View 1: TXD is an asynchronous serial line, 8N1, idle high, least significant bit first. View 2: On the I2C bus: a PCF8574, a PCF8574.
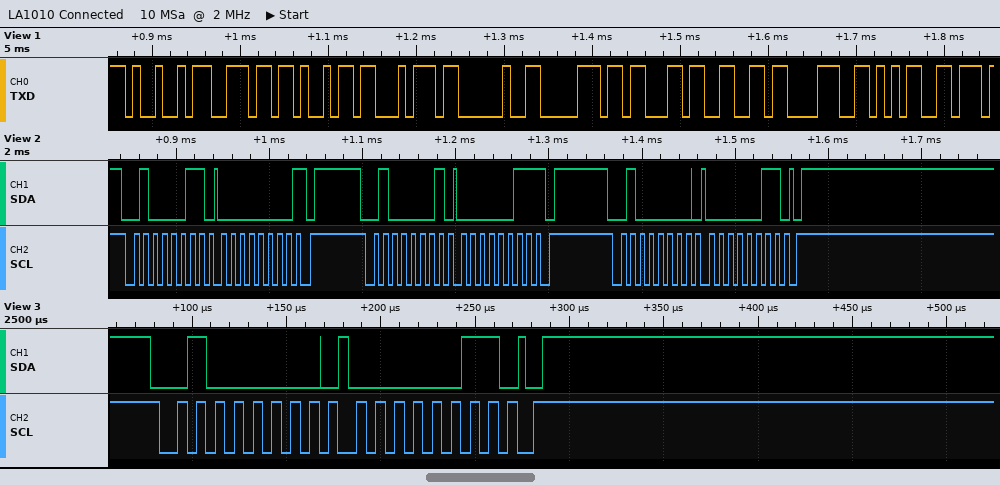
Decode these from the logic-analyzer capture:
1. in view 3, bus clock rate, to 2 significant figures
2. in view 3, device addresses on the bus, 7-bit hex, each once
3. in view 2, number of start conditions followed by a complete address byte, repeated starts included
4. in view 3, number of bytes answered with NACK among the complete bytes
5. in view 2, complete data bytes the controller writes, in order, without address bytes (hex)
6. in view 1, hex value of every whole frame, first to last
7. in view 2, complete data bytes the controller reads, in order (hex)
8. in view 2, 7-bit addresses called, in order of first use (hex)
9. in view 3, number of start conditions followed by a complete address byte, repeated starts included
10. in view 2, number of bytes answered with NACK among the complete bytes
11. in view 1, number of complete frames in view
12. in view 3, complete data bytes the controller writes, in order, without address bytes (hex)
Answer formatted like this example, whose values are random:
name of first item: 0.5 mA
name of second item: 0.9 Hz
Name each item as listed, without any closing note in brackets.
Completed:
in view 3, bus clock rate, to 2 significant figures: 100 kHz
in view 3, device addresses on the bus, 7-bit hex, each once: 0x20
in view 2, number of start conditions followed by a complete address byte, repeated starts included: 3
in view 3, number of bytes answered with NACK among the complete bytes: 0
in view 2, complete data bytes the controller writes, in order, without address bytes: 03
in view 1, hex value of every whole frame, first to last: 49 6E 69 74 20 70 63 66 38 35
in view 2, complete data bytes the controller reads, in order: 00 03
in view 2, 7-bit addresses called, in order of first use: 0x21 0x20
in view 3, number of start conditions followed by a complete address byte, repeated starts included: 1
in view 2, number of bytes answered with NACK among the complete bytes: 2
in view 1, number of complete frames in view: 10
in view 3, complete data bytes the controller writes, in order, without address bytes: 03
